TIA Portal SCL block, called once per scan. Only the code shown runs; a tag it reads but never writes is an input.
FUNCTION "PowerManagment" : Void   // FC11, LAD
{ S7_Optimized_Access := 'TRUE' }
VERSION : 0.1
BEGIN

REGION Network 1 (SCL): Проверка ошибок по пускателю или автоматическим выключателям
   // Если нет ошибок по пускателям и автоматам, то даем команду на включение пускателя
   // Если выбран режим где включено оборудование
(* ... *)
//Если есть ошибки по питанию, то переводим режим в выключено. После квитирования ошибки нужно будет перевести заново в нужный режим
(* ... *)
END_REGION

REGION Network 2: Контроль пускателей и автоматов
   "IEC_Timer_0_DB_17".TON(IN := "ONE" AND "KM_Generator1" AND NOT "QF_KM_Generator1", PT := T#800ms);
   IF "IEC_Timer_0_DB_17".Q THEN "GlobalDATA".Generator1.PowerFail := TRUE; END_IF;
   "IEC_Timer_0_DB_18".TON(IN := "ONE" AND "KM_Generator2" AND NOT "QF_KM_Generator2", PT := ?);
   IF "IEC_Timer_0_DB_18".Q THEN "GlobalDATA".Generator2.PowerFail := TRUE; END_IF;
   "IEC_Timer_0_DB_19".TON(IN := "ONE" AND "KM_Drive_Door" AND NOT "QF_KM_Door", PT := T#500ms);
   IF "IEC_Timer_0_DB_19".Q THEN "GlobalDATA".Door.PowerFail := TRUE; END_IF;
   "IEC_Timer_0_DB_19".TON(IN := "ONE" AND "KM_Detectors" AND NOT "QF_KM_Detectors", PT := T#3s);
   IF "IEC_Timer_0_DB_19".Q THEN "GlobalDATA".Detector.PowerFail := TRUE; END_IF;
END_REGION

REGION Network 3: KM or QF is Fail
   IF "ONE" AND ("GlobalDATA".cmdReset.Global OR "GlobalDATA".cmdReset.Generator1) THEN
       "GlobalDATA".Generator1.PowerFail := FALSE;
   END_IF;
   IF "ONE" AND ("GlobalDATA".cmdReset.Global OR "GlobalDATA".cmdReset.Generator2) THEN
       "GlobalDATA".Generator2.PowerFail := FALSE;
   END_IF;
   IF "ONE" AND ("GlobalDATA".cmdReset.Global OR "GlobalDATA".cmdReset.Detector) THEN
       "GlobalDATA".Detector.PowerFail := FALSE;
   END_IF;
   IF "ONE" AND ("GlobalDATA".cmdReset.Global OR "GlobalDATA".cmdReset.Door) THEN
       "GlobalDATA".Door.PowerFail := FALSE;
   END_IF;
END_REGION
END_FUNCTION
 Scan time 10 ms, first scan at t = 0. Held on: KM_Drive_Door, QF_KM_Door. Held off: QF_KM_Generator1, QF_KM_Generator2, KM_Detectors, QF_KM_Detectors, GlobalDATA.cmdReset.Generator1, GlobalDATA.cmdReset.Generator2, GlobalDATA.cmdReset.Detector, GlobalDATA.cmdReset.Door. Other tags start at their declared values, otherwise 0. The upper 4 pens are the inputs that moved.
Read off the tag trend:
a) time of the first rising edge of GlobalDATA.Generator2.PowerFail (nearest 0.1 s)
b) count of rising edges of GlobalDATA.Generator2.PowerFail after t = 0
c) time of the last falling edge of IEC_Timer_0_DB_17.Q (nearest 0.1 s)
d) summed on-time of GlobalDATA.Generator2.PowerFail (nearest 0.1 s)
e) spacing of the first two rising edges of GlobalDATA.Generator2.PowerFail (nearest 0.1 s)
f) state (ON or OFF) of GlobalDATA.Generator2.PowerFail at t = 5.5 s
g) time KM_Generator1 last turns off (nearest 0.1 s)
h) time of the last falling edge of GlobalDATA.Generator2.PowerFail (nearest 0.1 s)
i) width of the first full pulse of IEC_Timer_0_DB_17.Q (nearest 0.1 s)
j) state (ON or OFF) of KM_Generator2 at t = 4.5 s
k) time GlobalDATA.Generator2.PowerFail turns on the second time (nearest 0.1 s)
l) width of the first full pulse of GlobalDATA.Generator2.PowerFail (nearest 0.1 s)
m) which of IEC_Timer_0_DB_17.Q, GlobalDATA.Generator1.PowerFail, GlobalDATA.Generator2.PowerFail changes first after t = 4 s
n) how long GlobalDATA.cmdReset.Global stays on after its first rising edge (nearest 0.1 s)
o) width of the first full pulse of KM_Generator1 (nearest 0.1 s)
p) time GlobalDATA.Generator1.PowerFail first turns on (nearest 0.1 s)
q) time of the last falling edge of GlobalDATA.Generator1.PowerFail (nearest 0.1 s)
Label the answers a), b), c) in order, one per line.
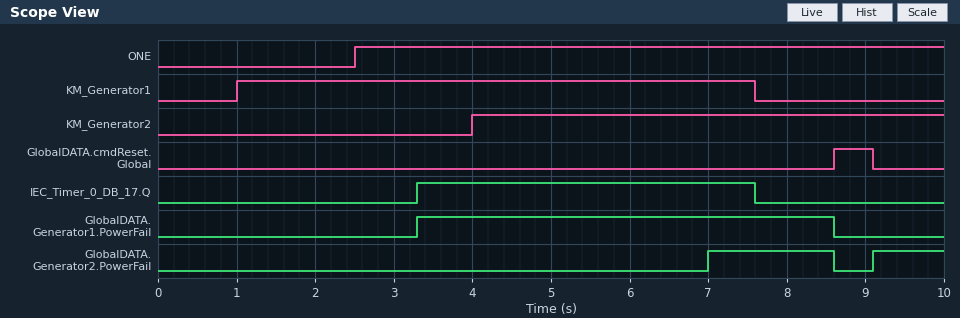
a) 7.0 s
b) 2
c) 7.6 s
d) 2.5 s
e) 2.1 s
f) OFF
g) 7.6 s
h) 8.6 s
i) 4.3 s
j) ON
k) 9.1 s
l) 1.6 s
m) GlobalDATA.Generator2.PowerFail
n) 0.5 s
o) 6.6 s
p) 3.3 s
q) 8.6 s
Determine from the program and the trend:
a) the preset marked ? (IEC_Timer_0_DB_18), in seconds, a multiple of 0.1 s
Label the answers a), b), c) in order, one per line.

a) 3.0 s
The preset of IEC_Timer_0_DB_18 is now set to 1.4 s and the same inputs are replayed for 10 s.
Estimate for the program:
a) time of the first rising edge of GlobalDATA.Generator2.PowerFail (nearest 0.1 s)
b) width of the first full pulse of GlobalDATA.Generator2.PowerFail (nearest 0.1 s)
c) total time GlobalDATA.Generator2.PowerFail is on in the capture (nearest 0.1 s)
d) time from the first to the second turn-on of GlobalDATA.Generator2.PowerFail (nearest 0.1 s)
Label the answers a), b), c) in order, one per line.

a) 5.4 s
b) 3.2 s
c) 4.1 s
d) 3.7 s
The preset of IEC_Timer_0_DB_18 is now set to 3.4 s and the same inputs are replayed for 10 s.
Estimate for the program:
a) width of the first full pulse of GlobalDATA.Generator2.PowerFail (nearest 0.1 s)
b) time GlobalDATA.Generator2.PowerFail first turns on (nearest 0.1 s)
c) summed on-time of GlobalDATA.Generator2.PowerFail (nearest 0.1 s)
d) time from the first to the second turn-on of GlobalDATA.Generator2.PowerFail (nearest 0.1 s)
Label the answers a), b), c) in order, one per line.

a) 1.2 s
b) 7.4 s
c) 2.1 s
d) 1.7 s
